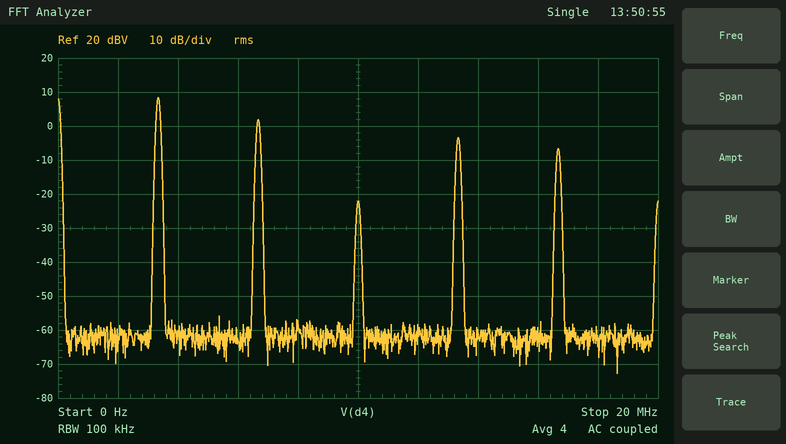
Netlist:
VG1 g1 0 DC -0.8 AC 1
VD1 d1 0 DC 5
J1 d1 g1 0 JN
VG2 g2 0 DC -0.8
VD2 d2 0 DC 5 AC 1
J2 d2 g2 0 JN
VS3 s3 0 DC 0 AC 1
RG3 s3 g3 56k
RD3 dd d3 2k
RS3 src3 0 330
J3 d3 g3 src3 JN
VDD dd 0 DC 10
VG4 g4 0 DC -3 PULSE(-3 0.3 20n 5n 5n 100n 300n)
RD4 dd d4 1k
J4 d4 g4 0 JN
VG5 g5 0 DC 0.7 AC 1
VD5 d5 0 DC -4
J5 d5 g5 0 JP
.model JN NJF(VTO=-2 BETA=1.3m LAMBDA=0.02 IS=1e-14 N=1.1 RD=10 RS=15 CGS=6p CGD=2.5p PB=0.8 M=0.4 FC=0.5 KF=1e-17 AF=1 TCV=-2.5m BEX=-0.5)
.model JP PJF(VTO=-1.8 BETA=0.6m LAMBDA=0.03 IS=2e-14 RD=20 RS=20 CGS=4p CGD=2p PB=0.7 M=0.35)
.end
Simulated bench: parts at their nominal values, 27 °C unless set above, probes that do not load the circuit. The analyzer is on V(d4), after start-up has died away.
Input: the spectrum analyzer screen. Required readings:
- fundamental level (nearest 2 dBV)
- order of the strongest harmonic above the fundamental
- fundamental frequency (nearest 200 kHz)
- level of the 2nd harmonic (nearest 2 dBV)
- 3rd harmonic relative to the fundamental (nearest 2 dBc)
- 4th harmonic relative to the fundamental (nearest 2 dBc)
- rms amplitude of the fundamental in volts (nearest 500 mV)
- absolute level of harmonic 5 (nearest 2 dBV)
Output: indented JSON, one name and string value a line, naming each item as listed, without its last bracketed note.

{
  "fundamental level": "8 dBV",
  "order of the strongest harmonic above the fundamental": "2",
  "fundamental frequency": "3.4 MHz",
  "level of the 2nd harmonic": "2 dBV",
  "3rd harmonic relative to the fundamental": "-30 dBc",
  "4th harmonic relative to the fundamental": "-12 dBc",
  "rms amplitude of the fundamental in volts": "2.5 V",
  "absolute level of harmonic 5": "-6 dBV"
}
